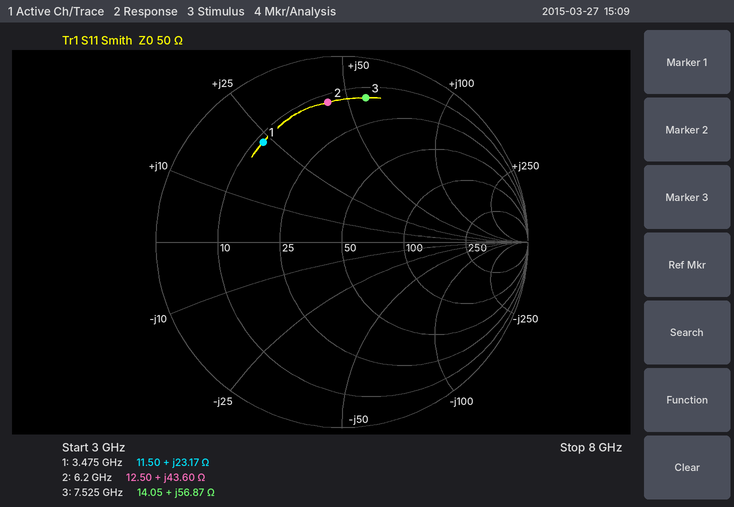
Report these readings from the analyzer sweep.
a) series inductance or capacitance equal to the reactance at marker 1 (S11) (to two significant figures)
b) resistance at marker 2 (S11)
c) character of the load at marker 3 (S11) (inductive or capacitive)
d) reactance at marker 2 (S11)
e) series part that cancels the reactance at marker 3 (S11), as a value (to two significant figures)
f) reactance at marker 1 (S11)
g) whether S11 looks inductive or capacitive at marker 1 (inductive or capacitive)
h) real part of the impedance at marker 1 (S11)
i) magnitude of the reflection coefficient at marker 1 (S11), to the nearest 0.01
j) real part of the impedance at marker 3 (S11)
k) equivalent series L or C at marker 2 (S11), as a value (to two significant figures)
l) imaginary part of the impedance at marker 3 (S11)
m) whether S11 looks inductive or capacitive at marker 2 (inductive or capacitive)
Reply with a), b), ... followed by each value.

a) 1.1 nH
b) 12.50 Ω
c) inductive
d) +43.60 Ω
e) 370 fF
f) +23.17 Ω
g) inductive
h) 11.50 Ω
i) 0.68
j) 14.05 Ω
k) 1.1 nH
l) +56.87 Ω
m) inductive
